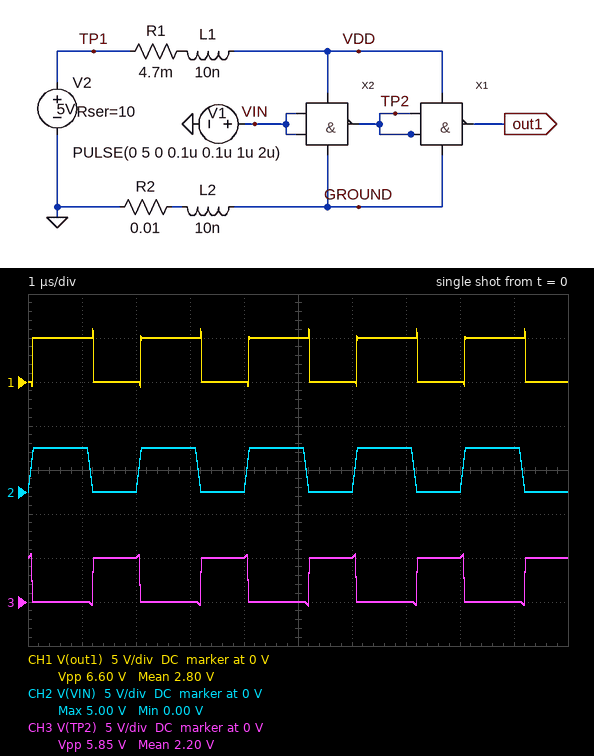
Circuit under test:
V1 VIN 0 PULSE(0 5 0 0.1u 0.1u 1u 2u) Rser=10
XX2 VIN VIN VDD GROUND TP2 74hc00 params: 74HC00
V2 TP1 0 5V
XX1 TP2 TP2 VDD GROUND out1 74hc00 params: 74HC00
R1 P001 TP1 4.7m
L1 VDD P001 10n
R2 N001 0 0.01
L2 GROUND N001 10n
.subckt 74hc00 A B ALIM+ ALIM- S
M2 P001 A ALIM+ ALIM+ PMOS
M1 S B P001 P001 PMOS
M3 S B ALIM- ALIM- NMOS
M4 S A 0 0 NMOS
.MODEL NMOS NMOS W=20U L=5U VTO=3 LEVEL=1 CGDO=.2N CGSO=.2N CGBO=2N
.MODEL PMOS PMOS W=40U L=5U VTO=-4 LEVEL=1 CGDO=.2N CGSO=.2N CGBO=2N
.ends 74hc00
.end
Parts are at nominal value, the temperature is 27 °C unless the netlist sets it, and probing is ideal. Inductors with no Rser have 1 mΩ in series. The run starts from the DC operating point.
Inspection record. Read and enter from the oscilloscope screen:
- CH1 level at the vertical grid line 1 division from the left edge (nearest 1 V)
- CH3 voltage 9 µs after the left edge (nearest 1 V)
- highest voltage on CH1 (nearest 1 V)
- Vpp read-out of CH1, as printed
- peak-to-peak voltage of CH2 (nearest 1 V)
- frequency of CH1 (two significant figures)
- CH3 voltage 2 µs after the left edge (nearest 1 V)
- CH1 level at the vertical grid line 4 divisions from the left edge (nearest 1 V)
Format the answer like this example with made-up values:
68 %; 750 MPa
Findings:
5 V; 0 V; 6 V; 6.60 V; 5 V; 500 kHz; 5 V; 0 V
